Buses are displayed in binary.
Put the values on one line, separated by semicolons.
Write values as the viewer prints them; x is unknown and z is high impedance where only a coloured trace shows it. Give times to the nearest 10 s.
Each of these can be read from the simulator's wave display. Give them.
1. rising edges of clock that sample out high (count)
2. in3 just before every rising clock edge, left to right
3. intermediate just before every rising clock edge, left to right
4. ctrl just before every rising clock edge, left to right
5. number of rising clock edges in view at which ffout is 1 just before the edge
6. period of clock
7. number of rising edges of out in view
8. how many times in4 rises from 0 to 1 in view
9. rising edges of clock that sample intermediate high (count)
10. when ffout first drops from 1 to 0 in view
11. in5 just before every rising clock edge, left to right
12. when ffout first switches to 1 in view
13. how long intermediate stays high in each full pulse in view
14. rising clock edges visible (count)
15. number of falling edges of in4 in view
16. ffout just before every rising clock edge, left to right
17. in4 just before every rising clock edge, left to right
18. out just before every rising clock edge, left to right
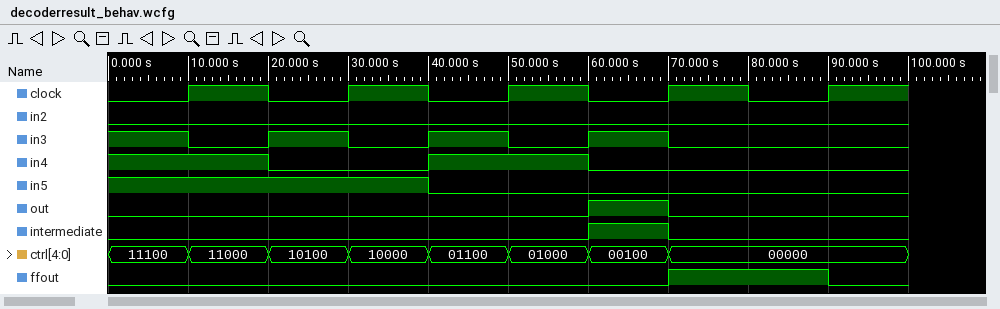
1; 1 1 1 1 0; 0 0 0 1 0; 11100, 10100, 01100, 00100, 00000; 1; 20 s; 1; 1; 1; 90 s; 1 1 0 0 0; 70 s; 10 s; 5; 2; 0 0 0 0 1; 1 0 1 0 0; 0 0 0 1 0
